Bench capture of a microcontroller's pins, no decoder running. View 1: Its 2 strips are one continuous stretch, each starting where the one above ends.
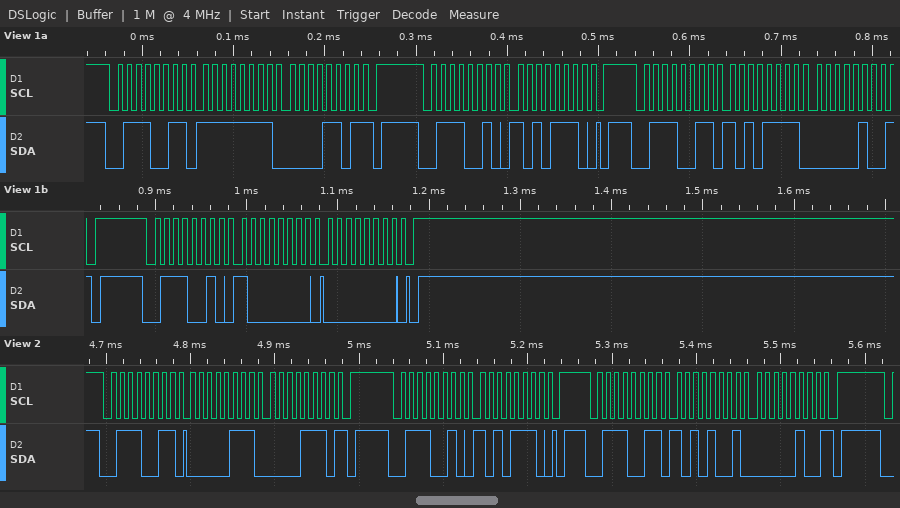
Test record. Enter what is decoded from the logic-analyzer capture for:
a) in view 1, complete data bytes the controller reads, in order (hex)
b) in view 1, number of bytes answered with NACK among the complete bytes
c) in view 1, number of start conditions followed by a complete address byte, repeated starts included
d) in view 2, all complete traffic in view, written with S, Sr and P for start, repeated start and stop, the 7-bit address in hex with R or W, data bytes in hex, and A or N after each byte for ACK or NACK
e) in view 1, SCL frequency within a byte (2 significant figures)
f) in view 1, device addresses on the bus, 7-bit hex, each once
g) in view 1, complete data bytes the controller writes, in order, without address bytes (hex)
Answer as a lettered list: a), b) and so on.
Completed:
a) FF 0D AF 04
b) 2
c) 4
d) S 39R A 07 A 0E N P S 39W A AE A P S 39R A A9 A 04 N P
e) 100 kHz
f) 0x39
g) AE 80 00
